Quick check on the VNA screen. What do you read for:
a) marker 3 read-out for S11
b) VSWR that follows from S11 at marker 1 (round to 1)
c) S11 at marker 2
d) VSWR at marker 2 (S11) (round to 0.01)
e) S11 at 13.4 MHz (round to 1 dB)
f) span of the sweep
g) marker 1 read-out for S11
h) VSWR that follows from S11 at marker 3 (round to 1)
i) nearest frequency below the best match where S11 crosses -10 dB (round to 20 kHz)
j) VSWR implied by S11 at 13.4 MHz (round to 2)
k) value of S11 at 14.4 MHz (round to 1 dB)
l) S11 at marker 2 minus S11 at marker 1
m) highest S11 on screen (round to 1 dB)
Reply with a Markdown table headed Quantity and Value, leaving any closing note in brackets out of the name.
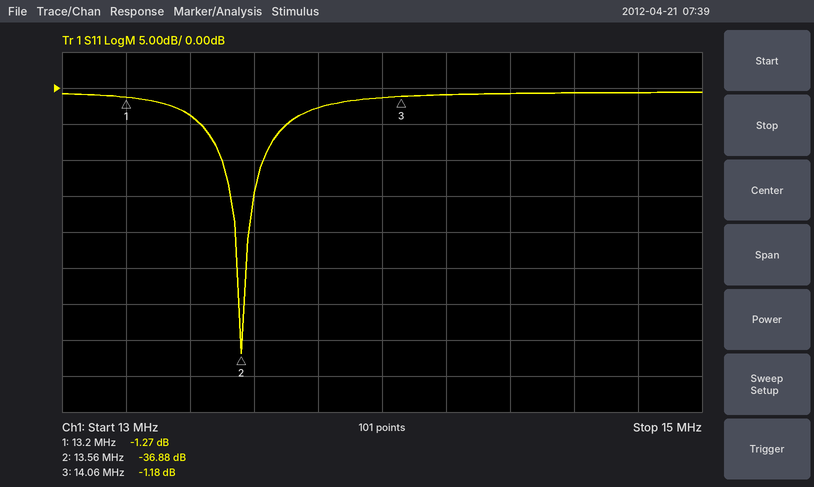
| Quantity | Value |
|---|---|
| marker 3 read-out for S11 | -1.18 dB |
| VSWR that follows from S11 at marker 1 | 14 |
| S11 at marker 2 | -36.88 dB |
| VSWR at marker 2 (S11) | 1.03 |
| S11 at 13.4 MHz | -4 dB |
| span of the sweep | 2 MHz |
| marker 1 read-out for S11 | -1.27 dB |
| VSWR that follows from S11 at marker 3 | 15 |
| nearest frequency below the best match where S11 crosses -10 dB | 13.50 MHz |
| VSWR implied by S11 at 13.4 MHz | 4 |
| value of S11 at 14.4 MHz | -1 dB |
| S11 at marker 2 minus S11 at marker 1 | -35.61 dB |
| highest S11 on screen | -1 dB |
